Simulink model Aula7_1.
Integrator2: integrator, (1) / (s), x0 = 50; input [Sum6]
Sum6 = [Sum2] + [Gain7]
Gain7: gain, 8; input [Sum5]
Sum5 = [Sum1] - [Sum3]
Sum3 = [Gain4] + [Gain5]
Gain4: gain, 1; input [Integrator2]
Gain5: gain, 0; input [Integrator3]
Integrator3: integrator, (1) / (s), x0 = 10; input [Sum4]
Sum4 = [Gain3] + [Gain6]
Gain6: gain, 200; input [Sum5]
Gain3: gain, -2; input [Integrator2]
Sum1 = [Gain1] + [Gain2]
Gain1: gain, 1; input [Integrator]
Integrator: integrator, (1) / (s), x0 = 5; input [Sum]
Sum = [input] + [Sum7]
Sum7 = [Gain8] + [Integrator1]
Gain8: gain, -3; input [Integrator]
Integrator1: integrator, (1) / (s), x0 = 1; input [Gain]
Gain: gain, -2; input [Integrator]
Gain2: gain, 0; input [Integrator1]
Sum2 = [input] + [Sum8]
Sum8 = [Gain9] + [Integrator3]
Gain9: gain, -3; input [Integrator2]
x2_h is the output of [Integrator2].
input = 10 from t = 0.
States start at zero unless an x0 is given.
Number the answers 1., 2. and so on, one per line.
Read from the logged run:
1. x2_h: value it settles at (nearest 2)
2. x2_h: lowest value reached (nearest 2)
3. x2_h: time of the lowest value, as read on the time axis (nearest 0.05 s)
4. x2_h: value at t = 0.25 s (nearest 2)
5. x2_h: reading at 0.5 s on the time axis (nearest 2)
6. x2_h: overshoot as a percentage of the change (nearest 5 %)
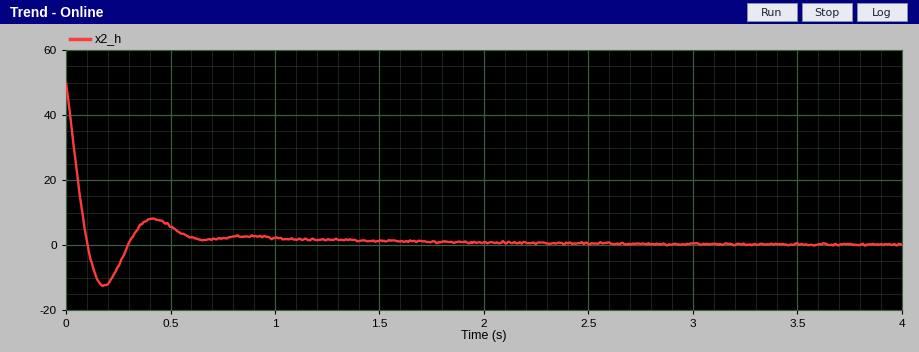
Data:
1. 0
2. -12
3. 0.20 s
4. -6
5. 6
6. 25 %
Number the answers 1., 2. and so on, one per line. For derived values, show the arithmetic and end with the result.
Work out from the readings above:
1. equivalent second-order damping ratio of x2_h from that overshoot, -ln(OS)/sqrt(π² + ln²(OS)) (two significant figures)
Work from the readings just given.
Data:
1. ln(0.25) = -1.386; 1.386 / sqrt(9.870 + 1.922) = 0.40
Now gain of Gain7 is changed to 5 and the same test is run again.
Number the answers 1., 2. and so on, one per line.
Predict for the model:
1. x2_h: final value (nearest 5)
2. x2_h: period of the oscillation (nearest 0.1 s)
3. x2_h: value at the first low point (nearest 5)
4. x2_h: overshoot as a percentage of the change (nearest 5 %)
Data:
1. 0
2. 0.5 s
3. -15
4. 35 %
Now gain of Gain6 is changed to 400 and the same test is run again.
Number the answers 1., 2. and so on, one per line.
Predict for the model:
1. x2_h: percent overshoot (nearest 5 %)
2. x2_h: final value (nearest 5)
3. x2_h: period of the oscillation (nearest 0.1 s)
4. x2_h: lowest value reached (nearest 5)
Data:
1. 35 %
2. 0
3. 0.3 s
4. -15
